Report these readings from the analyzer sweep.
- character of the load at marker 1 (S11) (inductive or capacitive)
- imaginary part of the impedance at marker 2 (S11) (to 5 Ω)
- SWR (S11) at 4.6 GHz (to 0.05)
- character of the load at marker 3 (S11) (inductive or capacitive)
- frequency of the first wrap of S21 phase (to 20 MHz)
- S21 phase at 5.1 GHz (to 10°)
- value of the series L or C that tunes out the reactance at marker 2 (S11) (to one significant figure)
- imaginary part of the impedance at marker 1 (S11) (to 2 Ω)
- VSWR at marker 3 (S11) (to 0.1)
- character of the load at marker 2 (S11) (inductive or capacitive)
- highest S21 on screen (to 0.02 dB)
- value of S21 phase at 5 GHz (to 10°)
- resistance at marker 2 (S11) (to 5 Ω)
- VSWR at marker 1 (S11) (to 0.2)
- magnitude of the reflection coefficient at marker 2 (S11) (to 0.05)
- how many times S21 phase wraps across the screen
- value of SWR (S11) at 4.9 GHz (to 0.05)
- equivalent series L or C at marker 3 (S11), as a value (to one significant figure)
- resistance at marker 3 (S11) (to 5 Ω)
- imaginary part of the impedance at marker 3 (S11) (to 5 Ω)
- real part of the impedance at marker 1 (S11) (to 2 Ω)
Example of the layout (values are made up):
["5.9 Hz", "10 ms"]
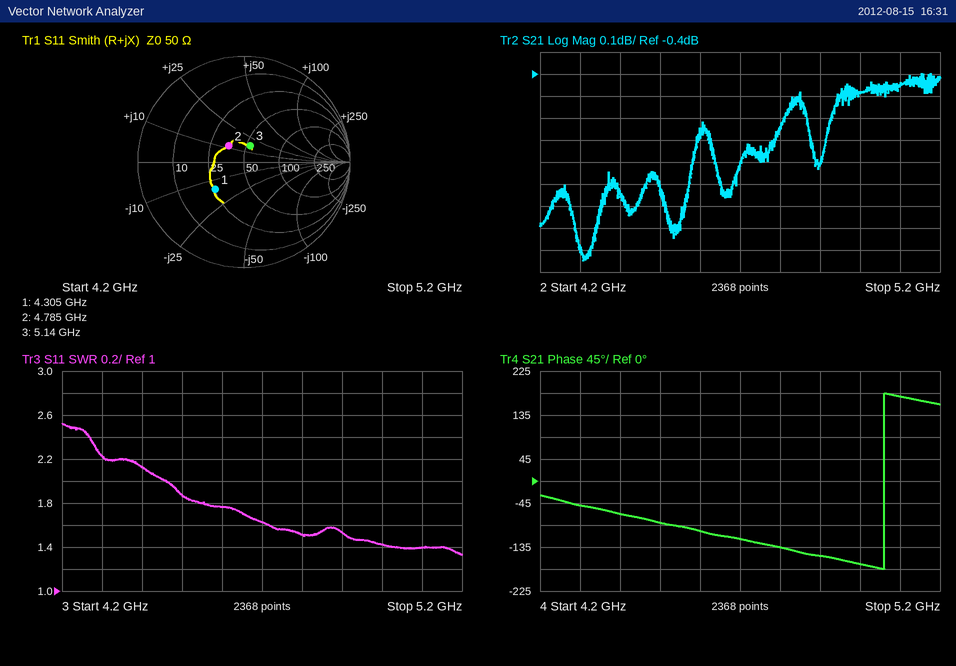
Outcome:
["capacitive", "+10 Ω", "1.75", "inductive", "5.06 GHz", "170°", "3 pF", "-16 Ω", "1.4", "inductive", "-0.40 dB", "-170°", "35 Ω", "2.2", "0.20", "1", "1.55", "500 pH", "55 Ω", "+15 Ω", "26 Ω"]
